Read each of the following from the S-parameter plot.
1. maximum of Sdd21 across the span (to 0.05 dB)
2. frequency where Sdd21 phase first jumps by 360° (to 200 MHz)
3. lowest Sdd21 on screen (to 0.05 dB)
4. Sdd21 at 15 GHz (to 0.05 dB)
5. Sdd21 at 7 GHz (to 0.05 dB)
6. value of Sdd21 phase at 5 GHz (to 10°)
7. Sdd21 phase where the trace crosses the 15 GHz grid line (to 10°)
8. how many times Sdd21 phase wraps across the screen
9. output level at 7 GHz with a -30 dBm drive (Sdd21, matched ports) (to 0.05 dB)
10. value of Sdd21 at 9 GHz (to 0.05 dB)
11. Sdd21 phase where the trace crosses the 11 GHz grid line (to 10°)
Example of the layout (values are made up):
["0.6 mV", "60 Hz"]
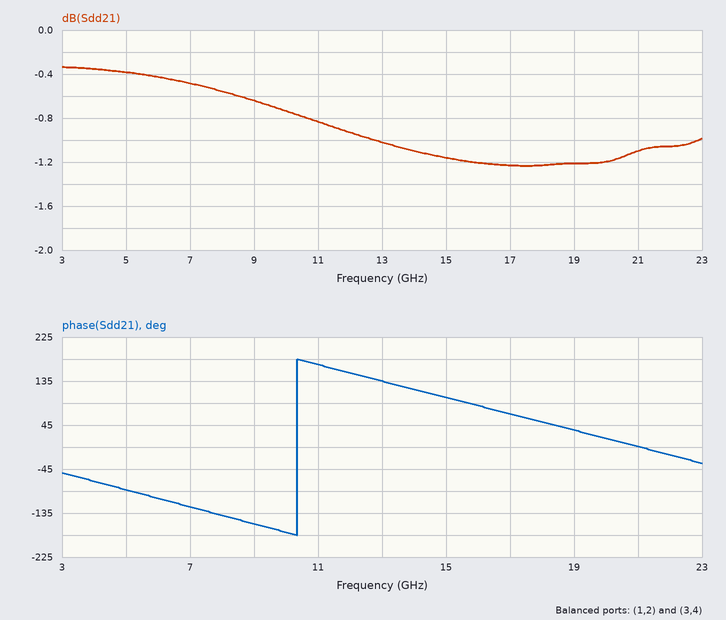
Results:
["-0.35 dB", "10.4 GHz", "-1.25 dB", "-1.15 dB", "-0.50 dB", "-90°", "100°", "1", "-30.50 dBm", "-0.65 dB", "170°"]
